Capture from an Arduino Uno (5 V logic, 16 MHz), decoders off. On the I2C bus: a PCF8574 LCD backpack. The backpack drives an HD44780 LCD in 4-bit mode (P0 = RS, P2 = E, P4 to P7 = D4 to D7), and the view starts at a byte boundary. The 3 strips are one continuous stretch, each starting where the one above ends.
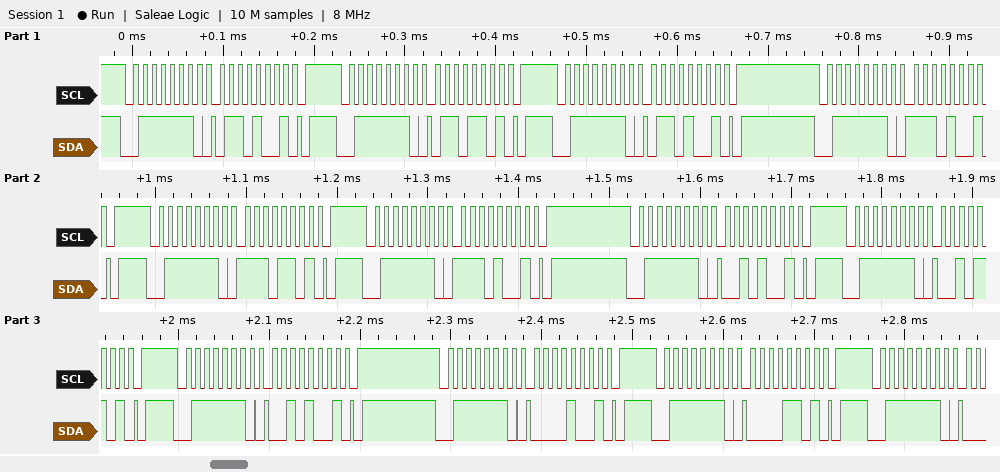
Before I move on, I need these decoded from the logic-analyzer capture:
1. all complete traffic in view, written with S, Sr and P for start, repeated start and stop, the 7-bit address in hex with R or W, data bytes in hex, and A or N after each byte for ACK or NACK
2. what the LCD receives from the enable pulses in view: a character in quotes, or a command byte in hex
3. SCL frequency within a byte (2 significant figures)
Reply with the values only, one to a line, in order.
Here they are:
S 3FW A 69 A P S 3FW A 6D A P S 3FW A 69 A P S 3FW A E9 A P S 3FW A ED A P S 3FW A E9 A P S 3FW A 29 A P S 3FW A 2D A P S 3FW A 29 A P S 3FW A 09 A P S 3FW A 0D A P S 3FW A
'n'
100 kHz
